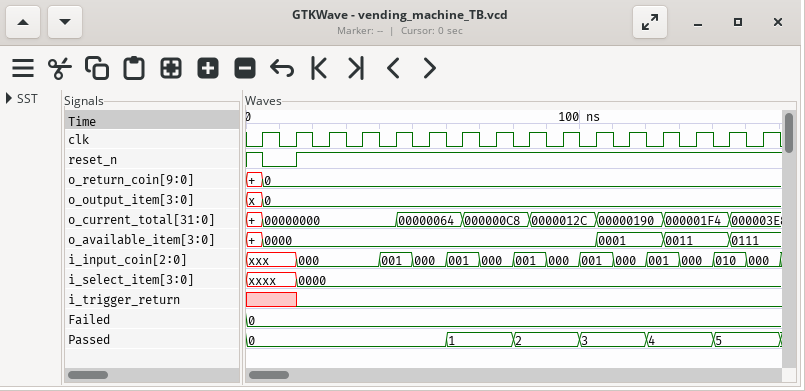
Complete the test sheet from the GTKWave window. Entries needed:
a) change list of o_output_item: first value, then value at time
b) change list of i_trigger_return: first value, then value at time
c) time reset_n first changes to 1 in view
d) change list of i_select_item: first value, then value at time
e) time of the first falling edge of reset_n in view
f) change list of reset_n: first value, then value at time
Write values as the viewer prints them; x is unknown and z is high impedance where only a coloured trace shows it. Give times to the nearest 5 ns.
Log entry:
x, 0 at 5 ns
x, 0 at 15 ns
15 ns
xxxx, 0000 at 15 ns
5 ns
1, 0 at 5 ns, 1 at 15 ns
